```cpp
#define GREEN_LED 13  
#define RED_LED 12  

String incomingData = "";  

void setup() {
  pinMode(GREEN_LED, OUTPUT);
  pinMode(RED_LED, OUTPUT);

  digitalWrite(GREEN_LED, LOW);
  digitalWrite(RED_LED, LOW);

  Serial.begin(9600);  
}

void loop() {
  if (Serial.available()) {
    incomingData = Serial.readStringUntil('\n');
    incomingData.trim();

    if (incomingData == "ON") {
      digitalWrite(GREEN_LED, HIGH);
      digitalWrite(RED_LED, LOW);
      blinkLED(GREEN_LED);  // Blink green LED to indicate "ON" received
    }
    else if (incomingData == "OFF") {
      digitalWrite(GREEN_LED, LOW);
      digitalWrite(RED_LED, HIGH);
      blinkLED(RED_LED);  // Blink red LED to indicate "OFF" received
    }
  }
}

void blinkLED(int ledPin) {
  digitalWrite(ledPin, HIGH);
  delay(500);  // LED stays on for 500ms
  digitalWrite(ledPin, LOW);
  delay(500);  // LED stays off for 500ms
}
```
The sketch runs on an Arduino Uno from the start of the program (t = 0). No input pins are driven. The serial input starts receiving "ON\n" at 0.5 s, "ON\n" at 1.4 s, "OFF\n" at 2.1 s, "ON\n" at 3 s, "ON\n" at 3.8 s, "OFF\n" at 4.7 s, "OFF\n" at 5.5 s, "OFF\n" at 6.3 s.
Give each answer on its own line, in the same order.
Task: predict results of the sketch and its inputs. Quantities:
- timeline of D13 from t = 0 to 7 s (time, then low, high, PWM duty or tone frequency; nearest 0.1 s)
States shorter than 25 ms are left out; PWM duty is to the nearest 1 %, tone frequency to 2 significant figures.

0 s low; 0.5 s high; 1 s low; 1.5 s high; 2 s low; 3.5 s high; 4 s low; 4.5 s high; 5 s low
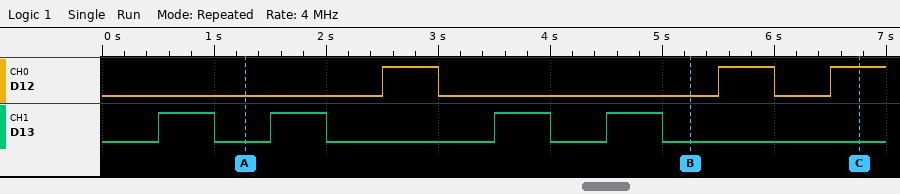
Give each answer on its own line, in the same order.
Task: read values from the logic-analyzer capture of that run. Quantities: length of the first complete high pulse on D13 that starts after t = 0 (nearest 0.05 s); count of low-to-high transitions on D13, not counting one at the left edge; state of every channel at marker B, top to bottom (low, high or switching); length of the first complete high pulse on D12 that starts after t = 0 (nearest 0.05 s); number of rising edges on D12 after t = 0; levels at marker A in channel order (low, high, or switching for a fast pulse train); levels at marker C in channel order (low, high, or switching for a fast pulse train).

0.50 s
4
D12 low, D13 low
0.50 s
3
D12 low, D13 low
D12 high, D13 low
